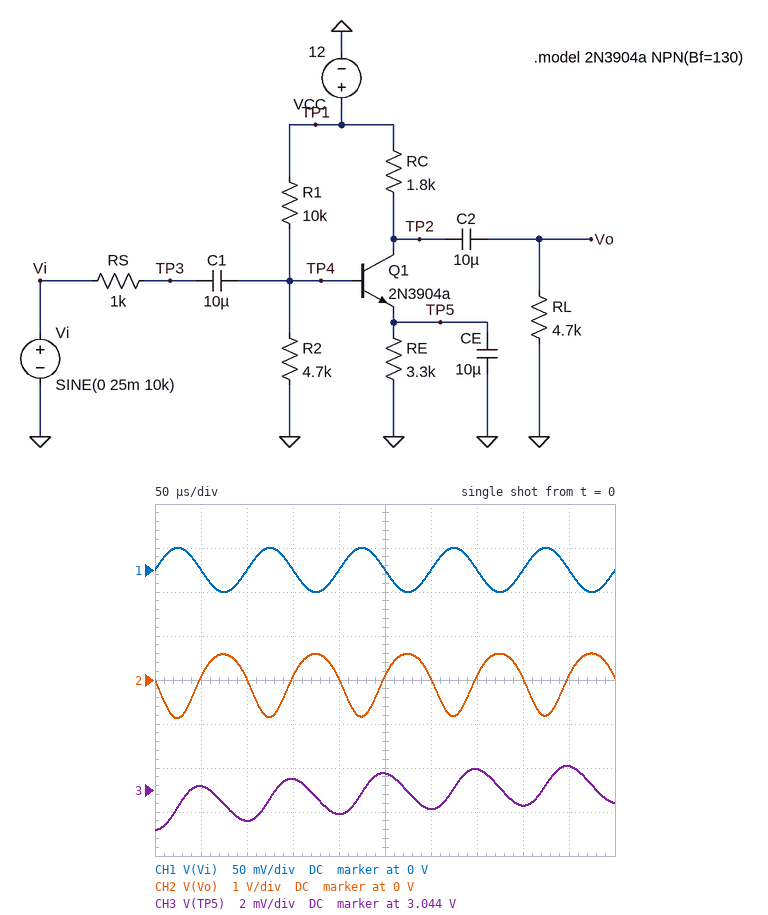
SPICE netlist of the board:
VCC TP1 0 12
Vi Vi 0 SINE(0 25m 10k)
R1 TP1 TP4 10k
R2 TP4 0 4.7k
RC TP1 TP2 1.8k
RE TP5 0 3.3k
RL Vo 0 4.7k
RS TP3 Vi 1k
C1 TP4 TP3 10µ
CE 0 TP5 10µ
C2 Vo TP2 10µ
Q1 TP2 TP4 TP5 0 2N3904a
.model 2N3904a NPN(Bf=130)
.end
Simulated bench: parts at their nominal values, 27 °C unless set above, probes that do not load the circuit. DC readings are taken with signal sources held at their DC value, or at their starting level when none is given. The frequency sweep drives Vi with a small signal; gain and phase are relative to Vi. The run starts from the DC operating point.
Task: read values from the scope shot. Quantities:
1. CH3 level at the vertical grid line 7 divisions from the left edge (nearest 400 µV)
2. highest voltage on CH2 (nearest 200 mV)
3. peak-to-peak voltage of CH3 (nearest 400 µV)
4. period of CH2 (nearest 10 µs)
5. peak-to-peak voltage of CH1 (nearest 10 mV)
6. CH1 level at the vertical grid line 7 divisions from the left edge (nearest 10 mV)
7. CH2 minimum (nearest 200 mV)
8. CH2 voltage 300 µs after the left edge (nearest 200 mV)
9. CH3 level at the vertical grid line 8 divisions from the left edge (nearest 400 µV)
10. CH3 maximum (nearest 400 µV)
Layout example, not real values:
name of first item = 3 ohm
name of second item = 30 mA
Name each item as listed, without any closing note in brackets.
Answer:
CH3 level at the vertical grid line 7 divisions from the left edge = 3.0448 V
highest voltage on CH2 = 600 mV
peak-to-peak voltage of CH3 = 2.8 mV
period of CH2 = 100 µs
peak-to-peak voltage of CH1 = 50 mV
CH1 level at the vertical grid line 7 divisions from the left edge = 0 V
CH2 minimum = -800 mV
CH2 voltage 300 µs after the left edge = 0 V
CH3 level at the vertical grid line 8 divisions from the left edge = 3.0432 V
CH3 maximum = 3.0452 V
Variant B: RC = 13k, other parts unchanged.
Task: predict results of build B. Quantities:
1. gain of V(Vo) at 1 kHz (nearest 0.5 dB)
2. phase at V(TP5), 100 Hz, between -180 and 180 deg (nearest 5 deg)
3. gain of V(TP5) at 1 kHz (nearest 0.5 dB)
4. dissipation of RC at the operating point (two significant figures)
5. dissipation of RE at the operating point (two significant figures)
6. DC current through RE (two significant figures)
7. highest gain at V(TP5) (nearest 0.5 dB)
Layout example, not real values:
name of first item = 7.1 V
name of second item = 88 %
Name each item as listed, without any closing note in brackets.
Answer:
gain of V(Vo) at 1 kHz = -15.0 dB
phase at V(TP5), 100 Hz, between -180 and 180 deg = -65 deg
gain of V(TP5) at 1 kHz = -36.0 dB
dissipation of RC at the operating point = 6.6 mW
dissipation of RE at the operating point = 2.2 mW
DC current through RE = 820 µA
highest gain at V(TP5) = -9.5 dB
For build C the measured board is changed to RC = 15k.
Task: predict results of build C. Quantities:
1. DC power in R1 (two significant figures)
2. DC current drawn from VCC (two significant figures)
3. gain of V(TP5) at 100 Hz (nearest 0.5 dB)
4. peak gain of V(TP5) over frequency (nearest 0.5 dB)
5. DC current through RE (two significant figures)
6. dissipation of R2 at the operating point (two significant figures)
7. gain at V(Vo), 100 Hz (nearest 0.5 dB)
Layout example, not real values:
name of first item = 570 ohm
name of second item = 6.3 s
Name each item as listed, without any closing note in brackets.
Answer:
DC power in R1 = 7.5 mW
DC current drawn from VCC = 1.5 mA
gain of V(TP5) at 100 Hz = -17.0 dB
peak gain of V(TP5) over frequency = -9.5 dB
DC current through RE = 780 µA
dissipation of R2 at the operating point = 2.4 mW
gain at V(Vo), 100 Hz = -15.5 dB
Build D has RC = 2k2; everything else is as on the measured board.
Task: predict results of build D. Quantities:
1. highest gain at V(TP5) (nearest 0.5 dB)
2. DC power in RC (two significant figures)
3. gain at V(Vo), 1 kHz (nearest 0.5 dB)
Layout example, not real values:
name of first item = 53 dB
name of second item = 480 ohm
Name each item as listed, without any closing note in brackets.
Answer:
highest gain at V(TP5) = -2.5 dB
DC power in RC = 1.8 mW
gain at V(Vo), 1 kHz = 29.5 dB
